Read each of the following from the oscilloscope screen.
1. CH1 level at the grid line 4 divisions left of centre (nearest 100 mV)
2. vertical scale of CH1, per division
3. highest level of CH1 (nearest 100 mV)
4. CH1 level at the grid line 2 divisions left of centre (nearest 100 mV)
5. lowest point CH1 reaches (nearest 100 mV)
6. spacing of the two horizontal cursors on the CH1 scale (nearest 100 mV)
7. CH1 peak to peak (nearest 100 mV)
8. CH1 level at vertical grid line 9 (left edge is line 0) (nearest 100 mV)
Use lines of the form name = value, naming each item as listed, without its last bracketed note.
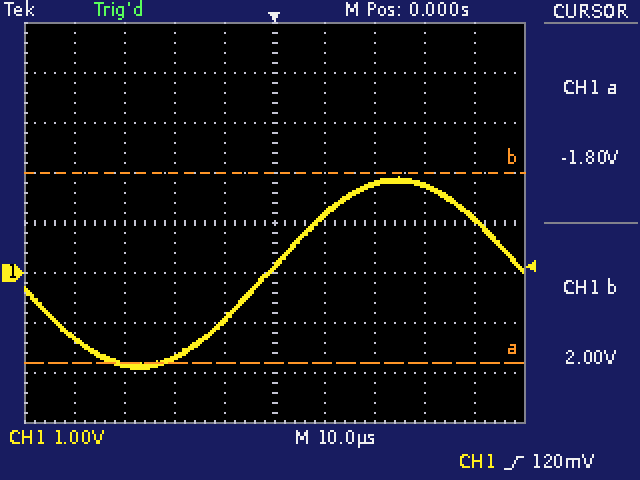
CH1 level at the grid line 4 divisions left of centre = -1.3 V
vertical scale of CH1, per division = 1 V
highest level of CH1 = 1.9 V
CH1 level at the grid line 2 divisions left of centre = -1.7 V
lowest point CH1 reaches = -1.9 V
spacing of the two horizontal cursors on the CH1 scale = 3.8 V
CH1 peak to peak = 3.8 V
CH1 level at vertical grid line 9 (left edge is line 0) = 1.1 V
